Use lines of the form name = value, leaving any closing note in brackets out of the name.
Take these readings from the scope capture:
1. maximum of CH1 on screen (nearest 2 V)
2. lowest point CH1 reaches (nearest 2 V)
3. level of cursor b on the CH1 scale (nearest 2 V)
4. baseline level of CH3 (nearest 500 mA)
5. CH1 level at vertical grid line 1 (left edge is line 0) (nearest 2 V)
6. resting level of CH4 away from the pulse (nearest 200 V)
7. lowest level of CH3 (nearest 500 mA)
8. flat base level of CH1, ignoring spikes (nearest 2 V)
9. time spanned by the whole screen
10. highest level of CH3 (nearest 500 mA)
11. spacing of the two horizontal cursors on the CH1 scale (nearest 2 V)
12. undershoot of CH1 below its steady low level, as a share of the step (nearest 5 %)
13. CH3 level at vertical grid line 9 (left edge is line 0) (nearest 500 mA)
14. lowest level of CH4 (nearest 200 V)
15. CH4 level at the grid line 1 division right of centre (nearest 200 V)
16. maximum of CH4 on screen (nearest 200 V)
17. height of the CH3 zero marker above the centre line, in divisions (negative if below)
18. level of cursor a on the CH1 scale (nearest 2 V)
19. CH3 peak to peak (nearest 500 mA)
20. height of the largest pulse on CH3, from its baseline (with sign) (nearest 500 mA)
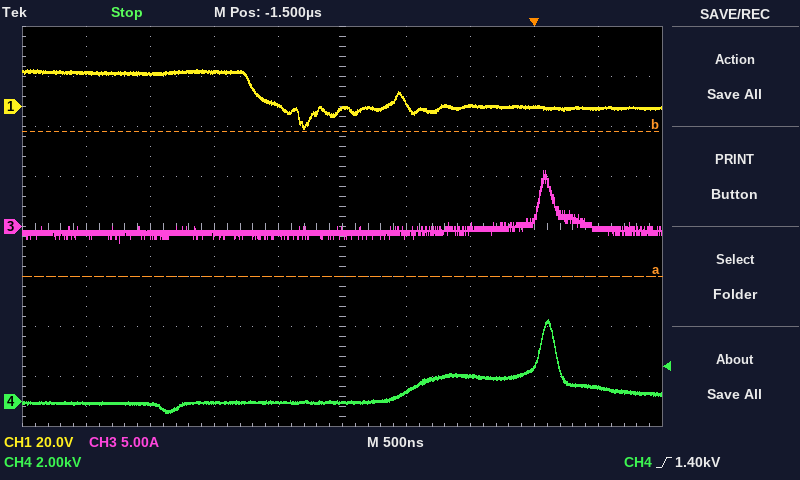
maximum of CH1 on screen = 14 V
lowest point CH1 reaches = -8 V
level of cursor b on the CH1 scale = -10 V
baseline level of CH3 = -500 mA
CH1 level at vertical grid line 1 (left edge is line 0) = 14 V
resting level of CH4 away from the pulse = 0.0 kV
lowest level of CH3 = -1.5 A
flat base level of CH1, ignoring spikes = 0 V
time spanned by the whole screen = 5 µs
highest level of CH3 = 5.5 A
spacing of the two horizontal cursors on the CH1 scale = 58 V
undershoot of CH1 below its steady low level, as a share of the step = 60 %
CH3 level at vertical grid line 9 (left edge is line 0) = 0.0 A
lowest level of CH4 = -400 V
CH4 level at the grid line 1 division right of centre = 400 V
maximum of CH4 on screen = 3.2 kV
height of the CH3 zero marker above the centre line, in divisions = 0.0 div
level of cursor a on the CH1 scale = -68 V
CH3 peak to peak = 7.0 A
height of the largest pulse on CH3, from its baseline (with sign) = +6.0 A
